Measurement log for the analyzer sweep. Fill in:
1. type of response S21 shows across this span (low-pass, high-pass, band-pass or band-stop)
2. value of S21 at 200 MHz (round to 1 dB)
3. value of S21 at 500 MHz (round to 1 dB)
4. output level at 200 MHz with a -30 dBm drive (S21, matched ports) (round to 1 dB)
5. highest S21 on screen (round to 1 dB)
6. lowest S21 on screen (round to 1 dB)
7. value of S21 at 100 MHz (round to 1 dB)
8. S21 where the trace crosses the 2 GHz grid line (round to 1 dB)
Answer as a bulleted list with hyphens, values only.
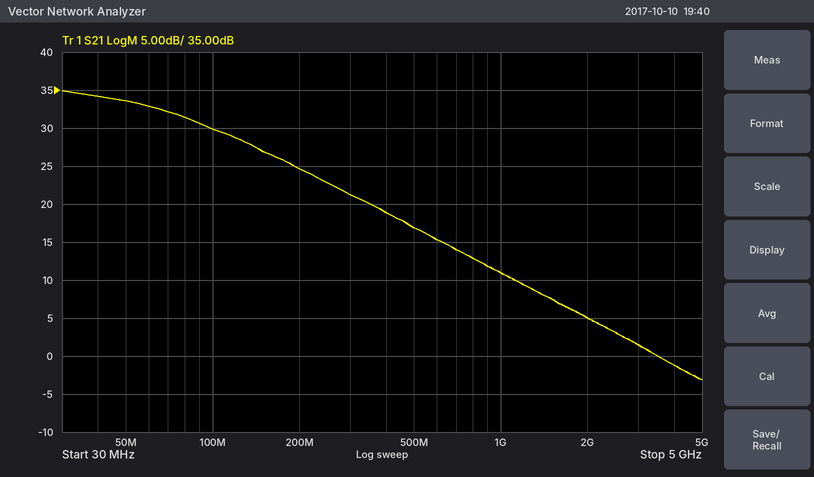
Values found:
- low-pass
- 25 dB
- 17 dB
- -5 dBm
- 35 dB
- -3 dB
- 30 dB
- 5 dB
